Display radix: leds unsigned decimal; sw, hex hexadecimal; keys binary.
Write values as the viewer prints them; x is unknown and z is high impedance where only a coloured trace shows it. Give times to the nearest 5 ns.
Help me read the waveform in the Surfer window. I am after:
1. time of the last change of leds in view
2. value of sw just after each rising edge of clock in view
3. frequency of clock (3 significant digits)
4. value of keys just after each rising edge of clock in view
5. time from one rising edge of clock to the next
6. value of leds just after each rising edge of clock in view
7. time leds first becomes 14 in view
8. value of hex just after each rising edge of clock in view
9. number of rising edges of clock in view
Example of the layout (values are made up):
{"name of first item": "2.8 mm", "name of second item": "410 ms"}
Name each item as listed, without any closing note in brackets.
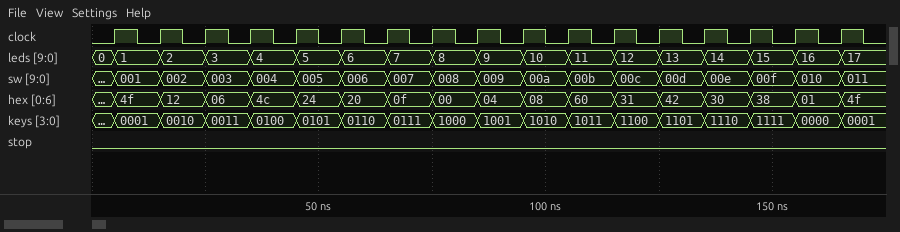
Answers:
{"time of the last change of leds in view": "165 ns", "value of sw just after each rising edge of clock in view": "001, 002, 003, 004, 005, 006, 007, 008, 009, 00a, 00b, 00c, 00d, 00e, 00f, 010, 011", "frequency of clock": "100 MHz", "value of keys just after each rising edge of clock in view": "0001, 0010, 0011, 0100, 0101, 0110, 0111, 1000, 1001, 1010, 1011, 1100, 1101, 1110, 1111, 0000, 0001", "time from one rising edge of clock to the next": "10 ns", "value of leds just after each rising edge of clock in view": "1, 2, 3, 4, 5, 6, 7, 8, 9, 10, 11, 12, 13, 14, 15, 16, 17", "time leds first becomes 14 in view": "135 ns", "value of hex just after each rising edge of clock in view": "4f, 12, 06, 4c, 24, 20, 0f, 00, 04, 08, 60, 31, 42, 30, 38, 01, 4f", "number of rising edges of clock in view": "17"}
